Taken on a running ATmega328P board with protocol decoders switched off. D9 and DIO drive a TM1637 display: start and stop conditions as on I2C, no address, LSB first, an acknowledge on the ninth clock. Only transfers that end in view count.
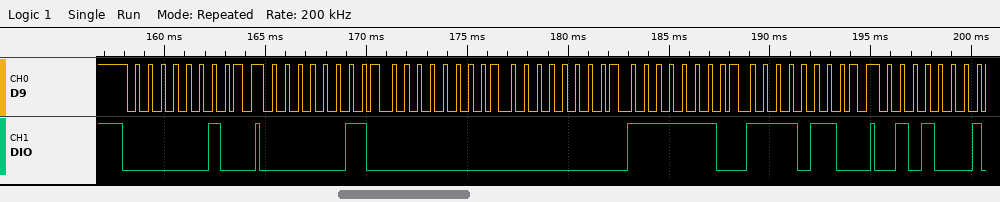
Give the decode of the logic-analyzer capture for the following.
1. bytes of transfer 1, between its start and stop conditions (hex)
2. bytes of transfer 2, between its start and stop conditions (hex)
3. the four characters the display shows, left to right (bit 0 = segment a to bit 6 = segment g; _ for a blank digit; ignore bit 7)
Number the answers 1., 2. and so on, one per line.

1. 40
2. C0 00 00 7F 6F
3. __89
